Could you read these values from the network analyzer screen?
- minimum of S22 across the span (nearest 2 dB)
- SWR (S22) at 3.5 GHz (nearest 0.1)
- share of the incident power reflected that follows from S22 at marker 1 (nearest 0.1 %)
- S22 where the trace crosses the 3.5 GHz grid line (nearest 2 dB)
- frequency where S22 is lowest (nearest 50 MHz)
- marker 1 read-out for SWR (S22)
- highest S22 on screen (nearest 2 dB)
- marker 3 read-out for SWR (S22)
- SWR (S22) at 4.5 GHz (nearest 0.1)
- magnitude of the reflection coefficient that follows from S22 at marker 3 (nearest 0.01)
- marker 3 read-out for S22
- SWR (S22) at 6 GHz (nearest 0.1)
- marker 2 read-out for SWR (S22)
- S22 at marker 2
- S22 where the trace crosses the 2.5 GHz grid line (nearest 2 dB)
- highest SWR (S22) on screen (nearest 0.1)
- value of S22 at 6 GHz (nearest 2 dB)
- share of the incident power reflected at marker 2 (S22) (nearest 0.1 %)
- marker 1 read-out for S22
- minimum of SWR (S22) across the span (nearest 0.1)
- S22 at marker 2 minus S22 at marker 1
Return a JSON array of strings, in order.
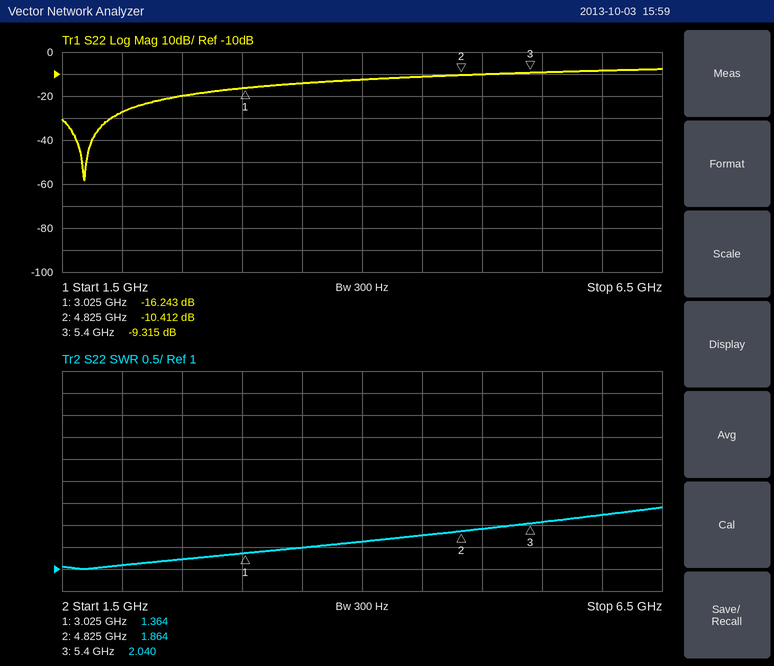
["-58 dB", "1.5", "2.4 %", "-14 dB", "1.70 GHz", "1.364", "-8 dB", "2.040", "1.8", "0.34", "-9.315 dB", "2.2", "1.864", "-10.412 dB", "-20 dB", "2.4", "-8 dB", "9.1 %", "-16.243 dB", "1.0", "5.831 dB"]
